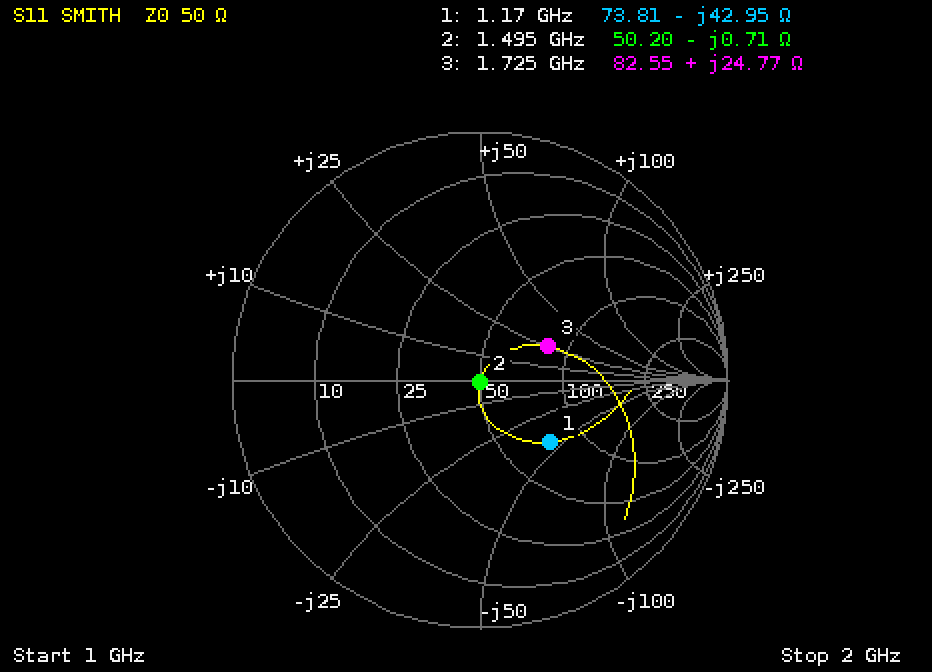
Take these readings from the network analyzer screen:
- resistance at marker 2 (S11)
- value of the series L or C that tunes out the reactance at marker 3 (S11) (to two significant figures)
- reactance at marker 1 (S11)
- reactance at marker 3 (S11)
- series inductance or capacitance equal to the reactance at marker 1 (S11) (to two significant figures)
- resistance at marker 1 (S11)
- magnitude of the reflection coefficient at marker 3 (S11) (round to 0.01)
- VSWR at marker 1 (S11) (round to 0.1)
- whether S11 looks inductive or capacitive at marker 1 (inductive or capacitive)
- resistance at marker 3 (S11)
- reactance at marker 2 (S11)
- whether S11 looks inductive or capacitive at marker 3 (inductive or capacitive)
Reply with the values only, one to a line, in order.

50.20 Ω
3.7 pF
-42.95 Ω
+24.77 Ω
3.2 pF
73.81 Ω
0.30
2.2
capacitive
82.55 Ω
-0.71 Ω
inductive
